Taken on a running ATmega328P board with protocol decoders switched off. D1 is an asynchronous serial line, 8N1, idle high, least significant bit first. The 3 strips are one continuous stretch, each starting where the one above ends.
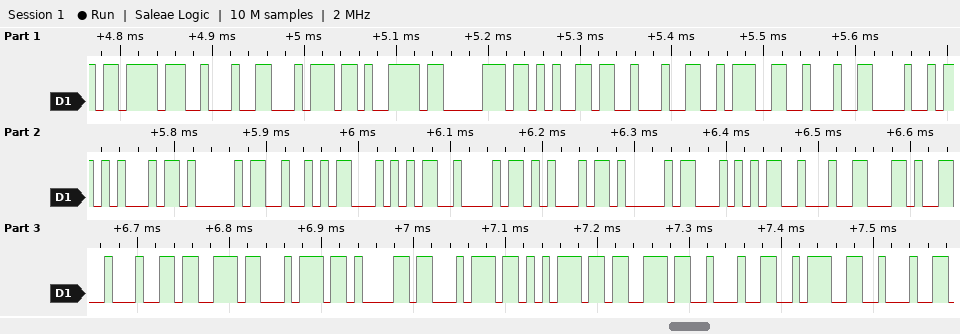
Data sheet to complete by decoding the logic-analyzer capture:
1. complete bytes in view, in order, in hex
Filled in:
0x7B 0x22 0x74 0x79 0x70 0x65 0x22 0x3A 0x22 0x48 0x45 0x41 0x52 0x54 0x42 0x45 0x41 0x54 0x22 0x2C 0x22 0x73 0x74 0x61 0x74 0x75 0x73 0x22 0x3A 0x22
